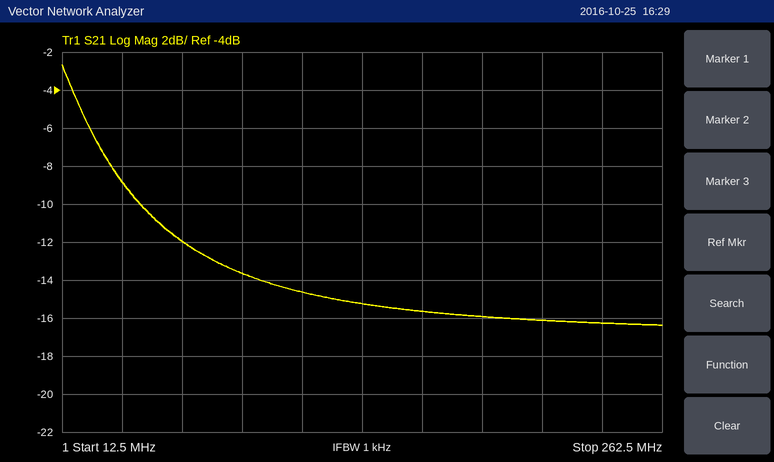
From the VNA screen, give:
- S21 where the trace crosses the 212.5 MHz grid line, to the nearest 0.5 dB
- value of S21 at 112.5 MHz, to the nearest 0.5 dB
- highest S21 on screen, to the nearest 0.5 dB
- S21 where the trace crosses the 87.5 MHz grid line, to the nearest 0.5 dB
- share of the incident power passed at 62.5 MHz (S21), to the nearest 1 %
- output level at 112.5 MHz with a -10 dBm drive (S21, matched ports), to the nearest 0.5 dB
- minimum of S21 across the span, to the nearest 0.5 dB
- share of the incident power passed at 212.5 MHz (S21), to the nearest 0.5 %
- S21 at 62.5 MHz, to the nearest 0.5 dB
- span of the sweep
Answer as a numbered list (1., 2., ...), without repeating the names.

1. -16.0 dB
2. -14.5 dB
3. -2.5 dB
4. -13.5 dB
5. 6 %
6. -24.5 dBm
7. -16.5 dB
8. 2.5 %
9. -12.0 dB
10. 250 MHz
